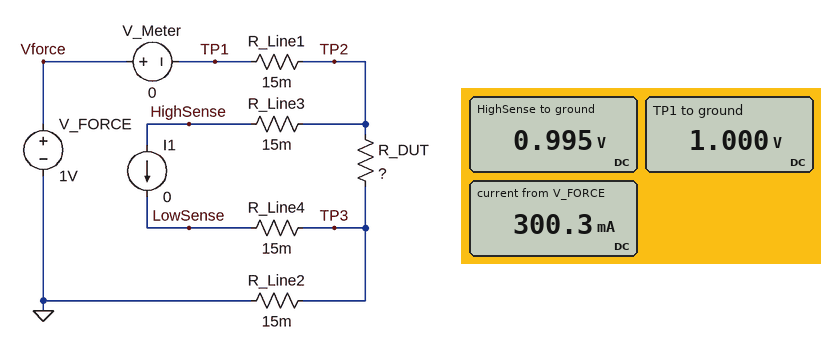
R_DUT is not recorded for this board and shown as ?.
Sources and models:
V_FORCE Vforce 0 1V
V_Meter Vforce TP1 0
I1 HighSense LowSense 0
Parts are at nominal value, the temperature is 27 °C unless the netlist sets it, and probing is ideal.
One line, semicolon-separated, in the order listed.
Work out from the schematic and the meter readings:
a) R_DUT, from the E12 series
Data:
3.3 Ω
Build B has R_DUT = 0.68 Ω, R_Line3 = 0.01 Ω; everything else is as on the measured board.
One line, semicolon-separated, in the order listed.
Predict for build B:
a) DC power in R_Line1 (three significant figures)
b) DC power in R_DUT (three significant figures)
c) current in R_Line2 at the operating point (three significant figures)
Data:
29.8 mW; 1.35 W; 1.41 A
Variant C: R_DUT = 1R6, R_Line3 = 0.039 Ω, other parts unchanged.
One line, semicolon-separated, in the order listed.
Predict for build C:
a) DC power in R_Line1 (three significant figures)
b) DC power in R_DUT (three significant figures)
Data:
5.65 mW; 602 mW
